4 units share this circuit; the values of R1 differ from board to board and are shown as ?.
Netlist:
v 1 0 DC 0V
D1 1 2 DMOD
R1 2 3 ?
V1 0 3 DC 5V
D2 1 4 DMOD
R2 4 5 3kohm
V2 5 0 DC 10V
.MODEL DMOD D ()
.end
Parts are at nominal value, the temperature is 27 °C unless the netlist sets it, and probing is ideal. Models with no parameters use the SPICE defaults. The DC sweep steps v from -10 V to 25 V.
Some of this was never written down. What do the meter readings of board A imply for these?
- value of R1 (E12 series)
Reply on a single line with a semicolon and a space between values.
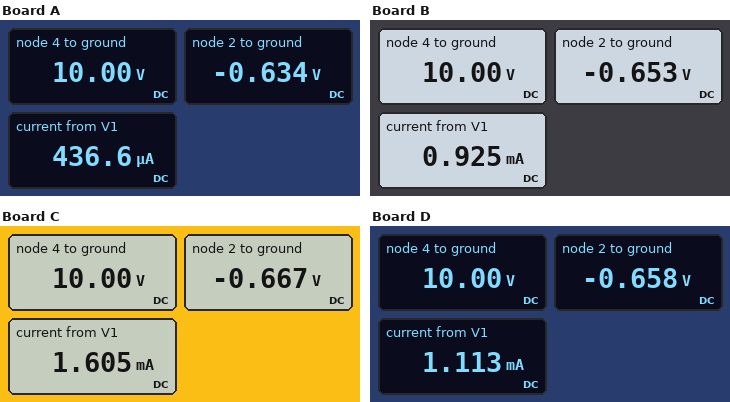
10 kΩ
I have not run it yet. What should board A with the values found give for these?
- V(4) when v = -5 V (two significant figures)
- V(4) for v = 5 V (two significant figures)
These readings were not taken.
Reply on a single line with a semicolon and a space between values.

10 V; 10 V
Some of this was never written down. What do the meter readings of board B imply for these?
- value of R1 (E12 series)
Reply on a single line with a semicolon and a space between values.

4.7 kΩ
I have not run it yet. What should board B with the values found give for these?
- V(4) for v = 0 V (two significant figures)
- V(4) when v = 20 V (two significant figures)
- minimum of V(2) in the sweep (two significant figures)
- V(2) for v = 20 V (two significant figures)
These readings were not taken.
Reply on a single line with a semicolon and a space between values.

10 V; 19 V; -5.0 V; 19 V
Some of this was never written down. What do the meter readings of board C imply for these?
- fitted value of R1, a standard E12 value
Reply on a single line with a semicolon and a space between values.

2.7 kΩ
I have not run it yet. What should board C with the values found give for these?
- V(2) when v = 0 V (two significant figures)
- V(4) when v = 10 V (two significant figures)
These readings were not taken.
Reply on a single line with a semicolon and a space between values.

-670 mV; 10 V
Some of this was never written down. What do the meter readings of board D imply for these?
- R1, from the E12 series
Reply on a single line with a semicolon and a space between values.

3.9 kΩ
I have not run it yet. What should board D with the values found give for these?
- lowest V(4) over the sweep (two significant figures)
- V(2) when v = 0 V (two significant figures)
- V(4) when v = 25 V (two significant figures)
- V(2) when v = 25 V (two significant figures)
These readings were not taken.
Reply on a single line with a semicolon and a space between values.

10 V; -660 mV; 24 V; 24 V
